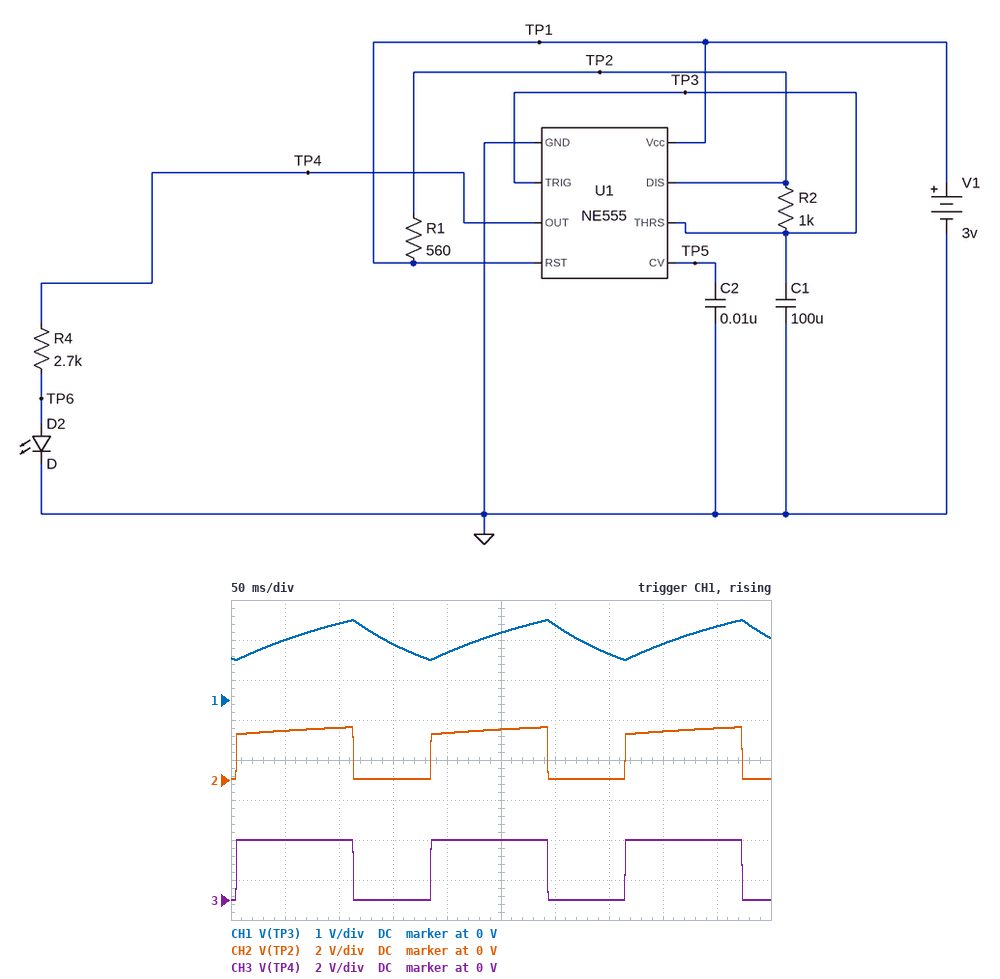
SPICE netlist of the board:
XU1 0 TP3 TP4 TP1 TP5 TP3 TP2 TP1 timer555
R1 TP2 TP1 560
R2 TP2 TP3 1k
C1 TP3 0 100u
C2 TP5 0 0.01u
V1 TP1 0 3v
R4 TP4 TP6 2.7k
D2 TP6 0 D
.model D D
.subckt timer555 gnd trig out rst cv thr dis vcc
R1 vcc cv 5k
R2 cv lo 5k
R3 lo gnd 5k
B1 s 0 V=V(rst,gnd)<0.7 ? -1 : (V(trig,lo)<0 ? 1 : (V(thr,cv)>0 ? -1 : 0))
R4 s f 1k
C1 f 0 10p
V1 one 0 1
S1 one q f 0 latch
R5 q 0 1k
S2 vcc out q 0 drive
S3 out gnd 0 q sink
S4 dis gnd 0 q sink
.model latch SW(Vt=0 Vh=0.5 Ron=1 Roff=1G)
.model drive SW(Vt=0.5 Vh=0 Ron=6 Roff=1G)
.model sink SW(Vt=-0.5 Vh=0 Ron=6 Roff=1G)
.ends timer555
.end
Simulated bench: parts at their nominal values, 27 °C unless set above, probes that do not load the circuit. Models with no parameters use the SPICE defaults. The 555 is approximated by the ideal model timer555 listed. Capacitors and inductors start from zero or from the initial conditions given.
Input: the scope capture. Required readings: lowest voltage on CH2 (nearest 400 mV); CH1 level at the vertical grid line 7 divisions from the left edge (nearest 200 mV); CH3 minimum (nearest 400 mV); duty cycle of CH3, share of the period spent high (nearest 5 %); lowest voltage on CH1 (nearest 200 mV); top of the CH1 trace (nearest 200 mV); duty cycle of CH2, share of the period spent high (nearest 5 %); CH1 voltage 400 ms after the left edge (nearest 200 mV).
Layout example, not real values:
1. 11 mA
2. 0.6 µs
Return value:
1. 0 V
2. 1.2 V
3. 0 V
4. 60 %
5. 1.0 V
6. 2.0 V
7. 60 %
8. 1.4 V
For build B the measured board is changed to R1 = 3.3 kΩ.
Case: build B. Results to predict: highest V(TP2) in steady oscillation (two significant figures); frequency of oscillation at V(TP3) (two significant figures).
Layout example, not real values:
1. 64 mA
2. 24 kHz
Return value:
1. 2.2 V
2. 2.7 Hz
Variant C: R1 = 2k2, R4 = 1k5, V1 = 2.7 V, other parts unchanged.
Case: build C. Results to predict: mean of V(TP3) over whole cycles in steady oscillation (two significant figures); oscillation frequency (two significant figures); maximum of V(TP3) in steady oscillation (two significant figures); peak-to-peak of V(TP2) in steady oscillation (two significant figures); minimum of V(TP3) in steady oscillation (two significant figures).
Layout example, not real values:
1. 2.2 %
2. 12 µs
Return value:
1. 1.4 V
2. 3.4 Hz
3. 1.8 V
4. 2.1 V
5. 900 mV
